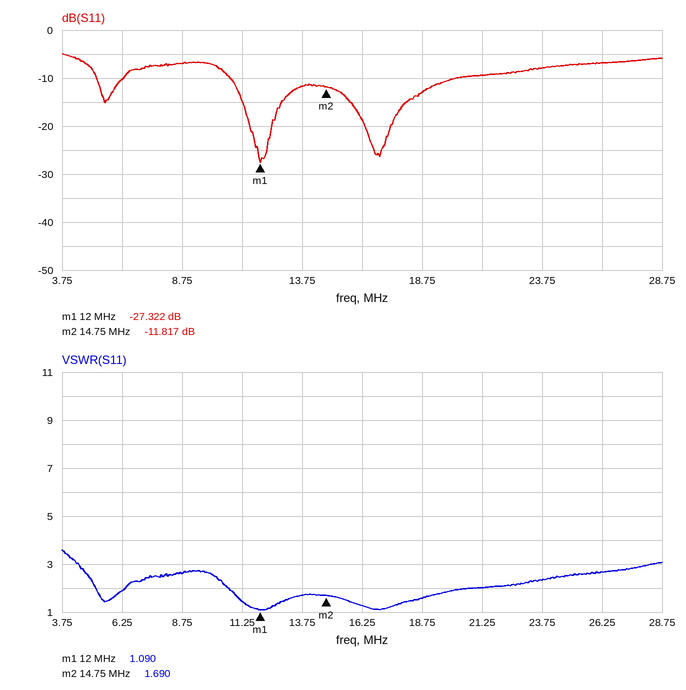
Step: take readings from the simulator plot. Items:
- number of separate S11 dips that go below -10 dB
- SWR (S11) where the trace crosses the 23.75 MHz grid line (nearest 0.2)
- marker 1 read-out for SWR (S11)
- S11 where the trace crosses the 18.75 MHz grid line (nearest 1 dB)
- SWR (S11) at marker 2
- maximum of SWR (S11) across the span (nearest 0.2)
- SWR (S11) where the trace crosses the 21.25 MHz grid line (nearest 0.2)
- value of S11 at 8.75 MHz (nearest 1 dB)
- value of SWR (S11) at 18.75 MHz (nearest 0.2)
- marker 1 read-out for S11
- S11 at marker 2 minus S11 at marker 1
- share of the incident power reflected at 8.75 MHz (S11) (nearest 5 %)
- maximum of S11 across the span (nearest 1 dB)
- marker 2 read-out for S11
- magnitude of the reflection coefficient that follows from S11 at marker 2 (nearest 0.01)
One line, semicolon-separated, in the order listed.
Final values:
3; 2.4; 1.090; -13 dB; 1.690; 3.6; 2.0; -7 dB; 1.6; -27.322 dB; 15.505 dB; 20 %; -5 dB; -11.817 dB; 0.26
